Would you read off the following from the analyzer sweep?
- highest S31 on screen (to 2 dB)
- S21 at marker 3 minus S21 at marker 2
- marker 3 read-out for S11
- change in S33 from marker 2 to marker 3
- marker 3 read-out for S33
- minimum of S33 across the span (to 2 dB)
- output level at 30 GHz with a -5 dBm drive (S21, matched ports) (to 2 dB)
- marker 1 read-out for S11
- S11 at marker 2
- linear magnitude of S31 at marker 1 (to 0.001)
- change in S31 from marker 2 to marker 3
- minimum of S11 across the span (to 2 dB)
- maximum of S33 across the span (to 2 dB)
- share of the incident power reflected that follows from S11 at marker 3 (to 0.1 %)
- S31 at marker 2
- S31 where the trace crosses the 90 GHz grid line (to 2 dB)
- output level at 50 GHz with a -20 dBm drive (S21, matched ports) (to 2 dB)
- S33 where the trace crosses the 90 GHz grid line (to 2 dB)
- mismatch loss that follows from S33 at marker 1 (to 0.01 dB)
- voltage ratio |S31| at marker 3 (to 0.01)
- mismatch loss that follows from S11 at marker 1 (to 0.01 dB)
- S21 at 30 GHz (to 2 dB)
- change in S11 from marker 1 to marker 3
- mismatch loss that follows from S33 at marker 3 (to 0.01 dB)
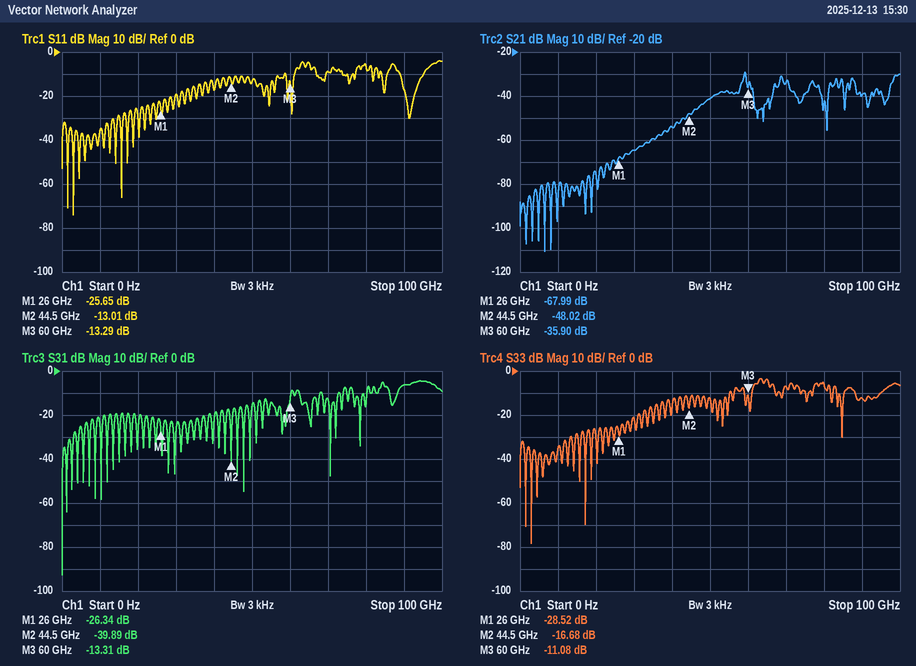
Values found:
-4 dB
12.12 dB
-13.29 dB
5.60 dB
-11.08 dB
-78 dB
-70 dBm
-25.65 dB
-13.01 dB
0.048
26.58 dB
-74 dB
-4 dB
4.7 %
-39.89 dB
-6 dB
-62 dBm
-12 dB
0.01 dB
0.22
0.01 dB
-64 dB
12.36 dB
0.35 dB
